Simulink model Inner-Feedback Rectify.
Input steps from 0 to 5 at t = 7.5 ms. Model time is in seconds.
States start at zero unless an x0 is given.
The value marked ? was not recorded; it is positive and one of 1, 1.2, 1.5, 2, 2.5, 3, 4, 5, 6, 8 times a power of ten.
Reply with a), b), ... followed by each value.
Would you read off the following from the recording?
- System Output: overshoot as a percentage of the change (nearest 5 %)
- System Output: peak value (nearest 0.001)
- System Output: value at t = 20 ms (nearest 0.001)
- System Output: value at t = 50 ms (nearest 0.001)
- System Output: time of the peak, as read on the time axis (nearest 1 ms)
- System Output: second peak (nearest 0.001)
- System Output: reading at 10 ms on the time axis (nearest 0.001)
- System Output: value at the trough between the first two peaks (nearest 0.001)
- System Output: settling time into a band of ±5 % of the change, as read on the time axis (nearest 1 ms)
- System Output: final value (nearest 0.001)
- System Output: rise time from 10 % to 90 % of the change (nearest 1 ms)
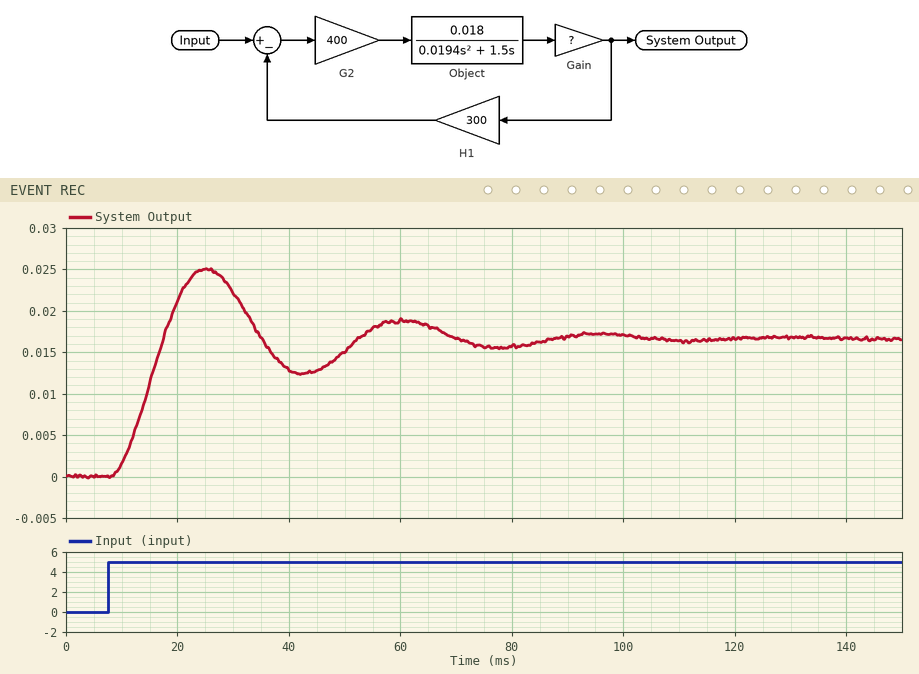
a) 50 %
b) 0.025
c) 0.021
d) 0.015
e) 25 ms
f) 0.019
g) 0.002
h) 0.012
i) 82 ms
j) 0.017
k) 7 ms
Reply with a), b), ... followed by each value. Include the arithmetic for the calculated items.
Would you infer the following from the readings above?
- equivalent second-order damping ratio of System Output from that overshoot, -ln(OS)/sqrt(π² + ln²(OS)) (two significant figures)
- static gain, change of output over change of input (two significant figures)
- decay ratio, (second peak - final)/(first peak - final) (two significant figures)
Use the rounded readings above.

a) ln(0.5) = -0.693; 0.693 / sqrt(9.870 + 0.480) = 0.22
b) (0.017 - 0) / (5 - 0) = 0.0034
c) (0.019 - 0.017) / (0.025 - 0.017) = 0.25
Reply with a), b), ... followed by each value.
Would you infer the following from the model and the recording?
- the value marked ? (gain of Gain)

a) 0.3
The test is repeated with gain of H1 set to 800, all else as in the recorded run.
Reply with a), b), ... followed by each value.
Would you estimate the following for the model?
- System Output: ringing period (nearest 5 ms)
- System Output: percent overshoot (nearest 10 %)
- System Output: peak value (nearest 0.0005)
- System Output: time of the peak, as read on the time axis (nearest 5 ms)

a) 20 ms
b) 70 %
c) 0.0105
d) 20 ms
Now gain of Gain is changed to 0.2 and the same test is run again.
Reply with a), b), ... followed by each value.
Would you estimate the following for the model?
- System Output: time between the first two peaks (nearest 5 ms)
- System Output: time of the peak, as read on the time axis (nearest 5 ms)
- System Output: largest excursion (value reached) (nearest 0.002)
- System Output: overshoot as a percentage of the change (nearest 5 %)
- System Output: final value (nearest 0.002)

a) 45 ms
b) 30 ms
c) 0.024
d) 45 %
e) 0.016
